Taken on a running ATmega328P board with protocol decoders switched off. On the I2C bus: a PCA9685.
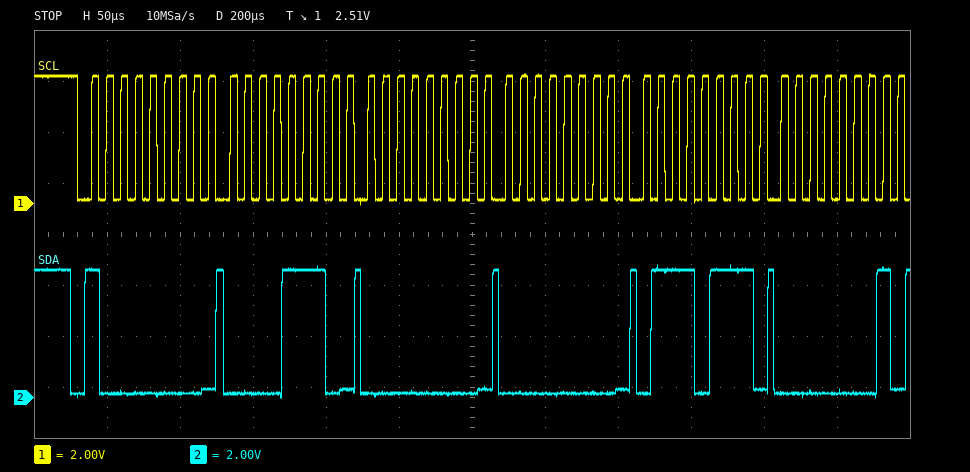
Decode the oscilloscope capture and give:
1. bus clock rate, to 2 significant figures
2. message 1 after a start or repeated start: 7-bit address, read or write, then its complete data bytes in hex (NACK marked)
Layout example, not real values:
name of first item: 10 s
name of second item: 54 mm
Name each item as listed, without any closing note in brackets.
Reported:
bus clock rate, to 2 significant figures: 100 kHz
message 1 after a start or repeated start: 7-bit address, read or write, then its complete data bytes in hex: 0x40 write: 0E 00 00 77 01
